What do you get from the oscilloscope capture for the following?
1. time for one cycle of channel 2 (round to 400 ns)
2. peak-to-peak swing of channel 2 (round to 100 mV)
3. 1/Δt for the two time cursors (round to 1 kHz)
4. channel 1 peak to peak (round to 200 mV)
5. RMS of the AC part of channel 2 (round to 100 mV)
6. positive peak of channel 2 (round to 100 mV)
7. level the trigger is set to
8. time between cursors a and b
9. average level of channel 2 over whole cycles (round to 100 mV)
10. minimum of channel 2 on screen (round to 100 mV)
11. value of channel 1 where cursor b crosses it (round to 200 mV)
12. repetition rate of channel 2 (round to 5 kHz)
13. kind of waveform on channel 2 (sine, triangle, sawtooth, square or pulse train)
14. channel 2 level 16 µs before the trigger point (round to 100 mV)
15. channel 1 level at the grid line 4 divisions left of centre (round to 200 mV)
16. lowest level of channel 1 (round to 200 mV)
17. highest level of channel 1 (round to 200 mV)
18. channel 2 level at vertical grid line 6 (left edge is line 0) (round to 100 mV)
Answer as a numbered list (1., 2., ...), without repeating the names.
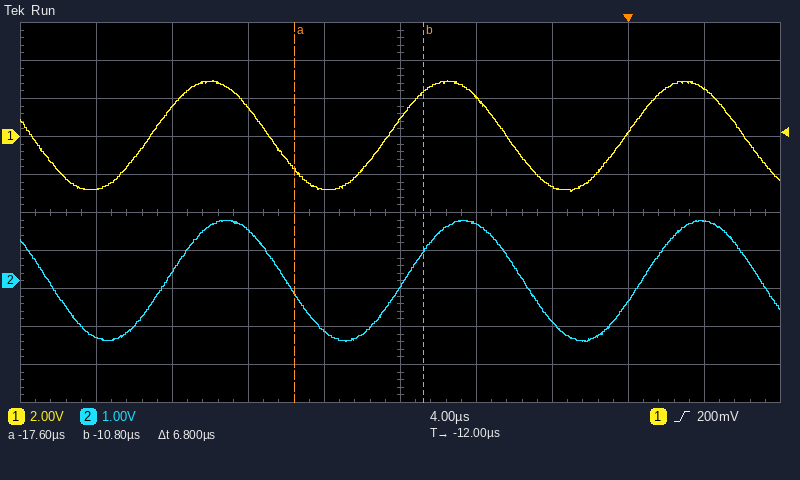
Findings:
1. 12.4 µs
2. 3.2 V
3. 147 kHz
4. 5.8 V
5. 1.1 V
6. 1.6 V
7. 200 mV
8. 6.8 µs
9. 0.0 V
10. -1.6 V
11. 2.4 V
12. 80 kHz
13. sine
14. -1.3 V
15. -2.8 V
16. -2.8 V
17. 3.0 V
18. 1.5 V
